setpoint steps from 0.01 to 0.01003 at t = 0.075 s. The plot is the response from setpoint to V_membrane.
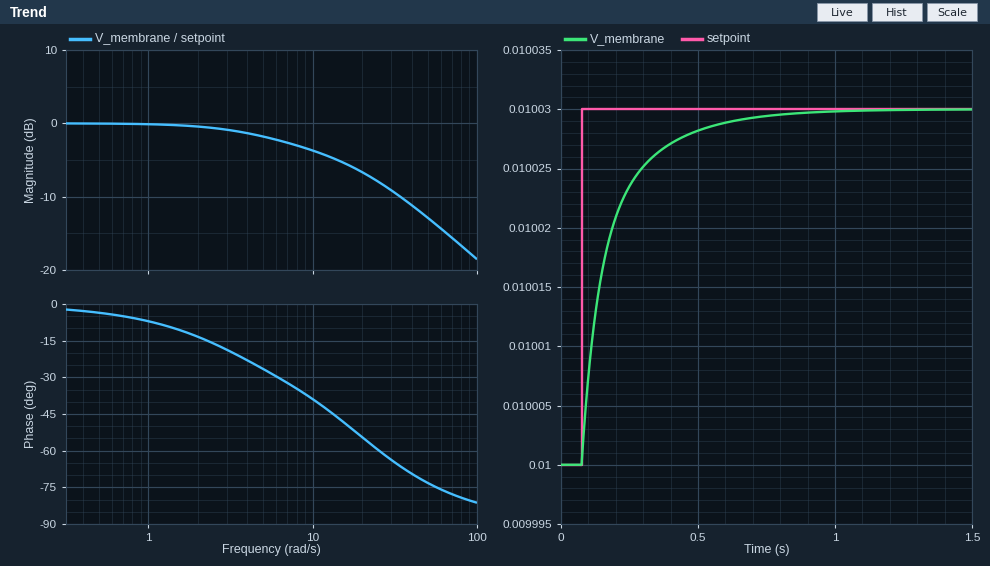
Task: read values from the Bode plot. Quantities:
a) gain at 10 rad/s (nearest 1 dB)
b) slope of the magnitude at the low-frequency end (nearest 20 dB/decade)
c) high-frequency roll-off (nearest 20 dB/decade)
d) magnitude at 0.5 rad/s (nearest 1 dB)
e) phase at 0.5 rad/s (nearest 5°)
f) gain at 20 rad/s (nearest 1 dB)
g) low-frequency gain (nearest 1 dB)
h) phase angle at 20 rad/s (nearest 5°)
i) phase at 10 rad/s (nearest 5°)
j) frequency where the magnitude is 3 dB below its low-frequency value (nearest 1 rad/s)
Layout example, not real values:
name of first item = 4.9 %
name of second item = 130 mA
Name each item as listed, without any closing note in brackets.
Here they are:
gain at 10 rad/s = -4 dB
slope of the magnitude at the low-frequency end = 0 dB/decade
high-frequency roll-off = -20 dB/decade
magnitude at 0.5 rad/s = 0 dB
phase at 0.5 rad/s = -5°
gain at 20 rad/s = -7 dB
low-frequency gain = 0 dB
phase angle at 20 rad/s = -55°
phase at 10 rad/s = -40°
frequency where the magnitude is 3 dB below its low-frequency value = 8 rad/s
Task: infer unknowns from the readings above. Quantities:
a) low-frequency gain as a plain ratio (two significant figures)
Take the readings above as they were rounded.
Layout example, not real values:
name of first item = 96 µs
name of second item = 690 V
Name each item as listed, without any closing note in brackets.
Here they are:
low-frequency gain as a plain ratio = 1.0
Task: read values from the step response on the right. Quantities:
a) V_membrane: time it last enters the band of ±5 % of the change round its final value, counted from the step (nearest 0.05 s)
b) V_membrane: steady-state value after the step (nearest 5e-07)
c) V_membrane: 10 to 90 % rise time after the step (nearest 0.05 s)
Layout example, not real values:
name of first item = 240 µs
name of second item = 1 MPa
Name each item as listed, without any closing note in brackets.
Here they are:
V_membrane: time it last enters the band of ±5 % of the change round its final value, counted from the step = 0.45 s
V_membrane: steady-state value after the step = 0.0100300
V_membrane: 10 to 90 % rise time after the step = 0.30 s
